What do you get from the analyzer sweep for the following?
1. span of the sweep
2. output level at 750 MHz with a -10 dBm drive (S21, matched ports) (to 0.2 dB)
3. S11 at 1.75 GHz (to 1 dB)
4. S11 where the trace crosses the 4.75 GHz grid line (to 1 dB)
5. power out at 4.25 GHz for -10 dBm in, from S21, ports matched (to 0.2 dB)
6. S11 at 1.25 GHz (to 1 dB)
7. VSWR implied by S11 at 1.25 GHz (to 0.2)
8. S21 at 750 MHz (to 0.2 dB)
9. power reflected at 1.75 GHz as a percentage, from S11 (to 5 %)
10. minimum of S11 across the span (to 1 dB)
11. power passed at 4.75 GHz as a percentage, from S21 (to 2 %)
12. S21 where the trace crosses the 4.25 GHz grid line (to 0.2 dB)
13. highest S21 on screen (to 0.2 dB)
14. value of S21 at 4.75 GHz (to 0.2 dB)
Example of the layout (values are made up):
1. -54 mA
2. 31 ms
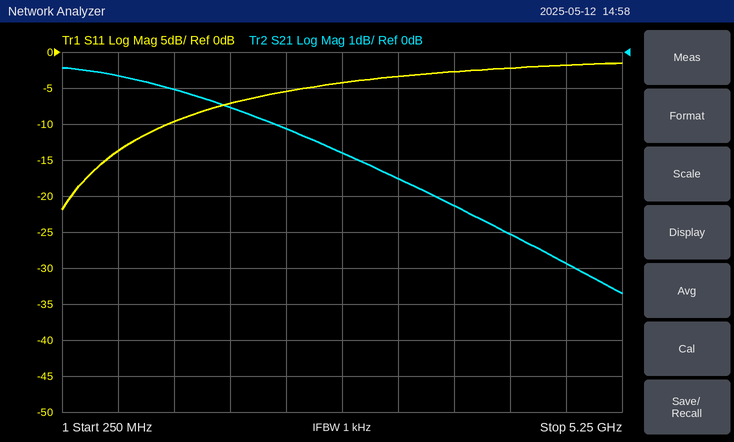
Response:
1. 5 GHz
2. -10.6 dBm
3. -7 dB
4. -2 dB
5. -15.0 dBm
6. -10 dB
7. 2.0
8. -0.6 dB
9. 20 %
10. -22 dB
11. 26 %
12. -5.0 dB
13. -0.4 dB
14. -5.8 dB
